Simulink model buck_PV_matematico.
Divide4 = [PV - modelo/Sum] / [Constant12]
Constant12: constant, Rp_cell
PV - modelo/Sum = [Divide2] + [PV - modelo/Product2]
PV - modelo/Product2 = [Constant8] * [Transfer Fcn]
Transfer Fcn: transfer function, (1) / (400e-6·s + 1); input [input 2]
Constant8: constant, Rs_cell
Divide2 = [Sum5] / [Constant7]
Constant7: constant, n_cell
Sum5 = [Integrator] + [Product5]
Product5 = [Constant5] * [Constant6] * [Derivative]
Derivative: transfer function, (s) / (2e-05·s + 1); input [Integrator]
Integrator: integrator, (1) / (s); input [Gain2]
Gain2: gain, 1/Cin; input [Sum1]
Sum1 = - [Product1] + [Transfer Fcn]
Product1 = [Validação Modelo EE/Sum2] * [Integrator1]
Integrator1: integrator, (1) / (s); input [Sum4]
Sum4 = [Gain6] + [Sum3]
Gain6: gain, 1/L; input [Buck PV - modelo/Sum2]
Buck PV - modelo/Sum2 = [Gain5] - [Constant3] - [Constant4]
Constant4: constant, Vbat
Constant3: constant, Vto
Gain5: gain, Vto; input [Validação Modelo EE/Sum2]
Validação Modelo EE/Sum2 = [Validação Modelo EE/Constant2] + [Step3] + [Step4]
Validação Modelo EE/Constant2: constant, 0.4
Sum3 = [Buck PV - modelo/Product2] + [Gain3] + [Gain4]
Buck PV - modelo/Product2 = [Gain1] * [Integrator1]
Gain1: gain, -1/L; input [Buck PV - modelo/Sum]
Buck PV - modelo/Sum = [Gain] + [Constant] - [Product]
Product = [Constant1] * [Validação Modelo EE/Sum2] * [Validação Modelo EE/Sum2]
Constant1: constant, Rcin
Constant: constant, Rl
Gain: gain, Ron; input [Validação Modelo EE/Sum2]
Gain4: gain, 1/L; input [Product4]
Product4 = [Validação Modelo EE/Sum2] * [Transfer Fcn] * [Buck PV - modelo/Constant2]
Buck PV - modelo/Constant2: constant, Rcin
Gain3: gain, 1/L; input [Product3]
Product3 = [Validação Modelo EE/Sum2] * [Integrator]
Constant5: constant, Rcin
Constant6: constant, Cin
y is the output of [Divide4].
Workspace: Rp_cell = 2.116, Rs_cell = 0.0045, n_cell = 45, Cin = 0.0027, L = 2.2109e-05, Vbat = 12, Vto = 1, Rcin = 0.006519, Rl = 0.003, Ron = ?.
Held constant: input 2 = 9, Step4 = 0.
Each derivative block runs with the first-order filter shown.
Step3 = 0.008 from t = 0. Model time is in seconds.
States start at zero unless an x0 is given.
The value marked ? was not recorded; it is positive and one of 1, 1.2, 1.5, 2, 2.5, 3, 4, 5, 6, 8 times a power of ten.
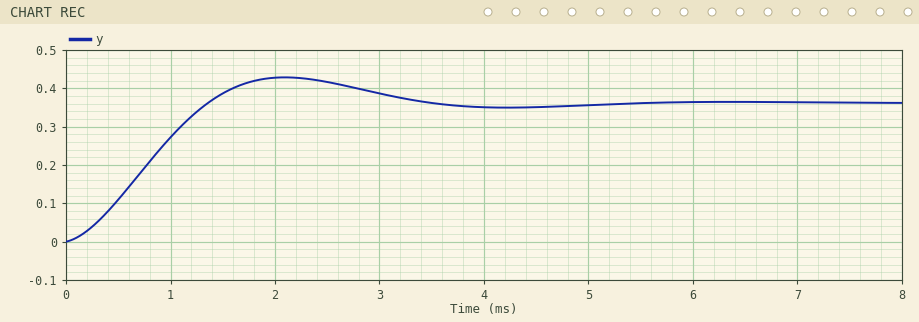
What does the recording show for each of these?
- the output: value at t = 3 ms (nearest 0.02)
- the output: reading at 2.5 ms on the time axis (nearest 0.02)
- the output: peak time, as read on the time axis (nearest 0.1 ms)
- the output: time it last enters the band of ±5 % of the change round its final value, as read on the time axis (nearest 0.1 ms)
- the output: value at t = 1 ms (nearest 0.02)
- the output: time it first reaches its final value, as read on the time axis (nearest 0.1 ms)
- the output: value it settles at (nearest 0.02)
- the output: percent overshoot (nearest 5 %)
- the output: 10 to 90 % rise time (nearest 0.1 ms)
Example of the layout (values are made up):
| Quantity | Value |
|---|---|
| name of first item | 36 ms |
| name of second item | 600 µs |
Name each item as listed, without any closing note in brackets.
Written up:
| Quantity | Value |
|---|---|
| the output: value at t = 3 ms | 0.38 |
| the output: reading at 2.5 ms on the time axis | 0.42 |
| the output: peak time, as read on the time axis | 2.1 ms |
| the output: time it last enters the band of ±5 % of the change round its final value, as read on the time axis | 3.1 ms |
| the output: value at t = 1 ms | 0.28 |
| the output: time it first reaches its final value, as read on the time axis | 1.4 ms |
| the output: value it settles at | 0.36 |
| the output: percent overshoot | 20 % |
| the output: 10 to 90 % rise time | 1.0 ms |
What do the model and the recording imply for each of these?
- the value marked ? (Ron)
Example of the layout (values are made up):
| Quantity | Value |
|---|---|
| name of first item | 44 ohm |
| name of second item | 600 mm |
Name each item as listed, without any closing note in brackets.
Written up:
| Quantity | Value |
|---|---|
| the value marked ? | 0.08 |
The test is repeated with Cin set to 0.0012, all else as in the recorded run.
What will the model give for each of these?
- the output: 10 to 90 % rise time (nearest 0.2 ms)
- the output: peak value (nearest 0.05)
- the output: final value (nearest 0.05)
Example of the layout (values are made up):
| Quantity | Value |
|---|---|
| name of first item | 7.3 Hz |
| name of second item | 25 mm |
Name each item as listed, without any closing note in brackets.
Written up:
| Quantity | Value |
|---|---|
| the output: 10 to 90 % rise time | 0.6 ms |
| the output: peak value | 0.50 |
| the output: final value | 0.35 |
